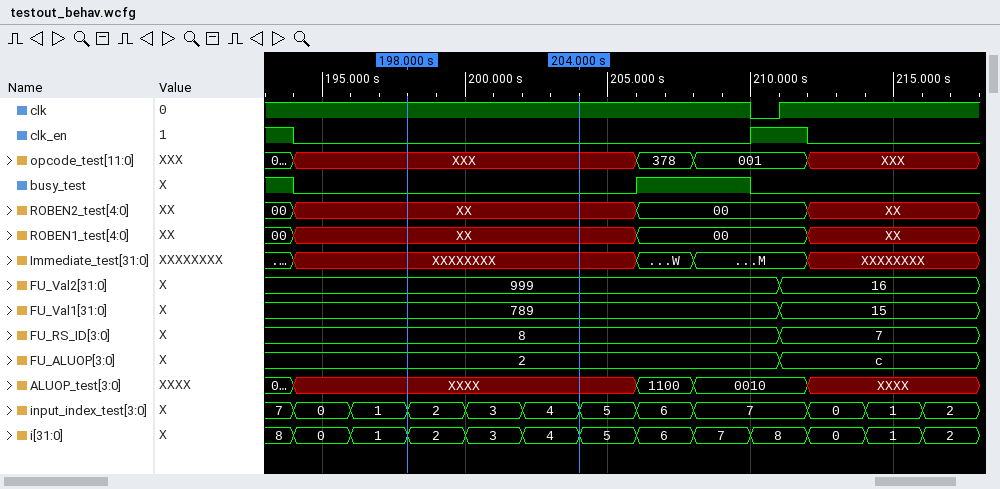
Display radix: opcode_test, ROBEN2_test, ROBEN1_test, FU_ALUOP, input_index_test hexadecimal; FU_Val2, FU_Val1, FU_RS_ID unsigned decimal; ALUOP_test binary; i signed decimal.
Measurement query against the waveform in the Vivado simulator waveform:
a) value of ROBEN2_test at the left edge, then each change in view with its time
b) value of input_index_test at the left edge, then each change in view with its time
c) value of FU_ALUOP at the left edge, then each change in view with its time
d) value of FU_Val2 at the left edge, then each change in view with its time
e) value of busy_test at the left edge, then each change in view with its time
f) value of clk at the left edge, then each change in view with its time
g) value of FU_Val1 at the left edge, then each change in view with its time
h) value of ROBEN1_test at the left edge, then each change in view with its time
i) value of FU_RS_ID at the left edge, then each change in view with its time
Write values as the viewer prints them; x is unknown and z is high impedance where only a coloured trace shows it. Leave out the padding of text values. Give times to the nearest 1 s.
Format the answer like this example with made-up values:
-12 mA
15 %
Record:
00, XX at 194 s, 00 at 206 s, XX at 212 s
7, 0 at 194 s, 1 at 196 s, 2 at 198 s, 3 at 200 s, 4 at 202 s, 5 at 204 s, 6 at 206 s, 7 at 208 s, 0 at 212 s, 1 at 214 s, 2 at 216 s
2, c at 211 s
999, 16 at 211 s
1, 0 at 194 s, 1 at 206 s, 0 at 210 s
1, 0 at 210 s, 1 at 211 s
789, 15 at 211 s
00, XX at 194 s, 00 at 206 s, XX at 212 s
8, 7 at 211 s
